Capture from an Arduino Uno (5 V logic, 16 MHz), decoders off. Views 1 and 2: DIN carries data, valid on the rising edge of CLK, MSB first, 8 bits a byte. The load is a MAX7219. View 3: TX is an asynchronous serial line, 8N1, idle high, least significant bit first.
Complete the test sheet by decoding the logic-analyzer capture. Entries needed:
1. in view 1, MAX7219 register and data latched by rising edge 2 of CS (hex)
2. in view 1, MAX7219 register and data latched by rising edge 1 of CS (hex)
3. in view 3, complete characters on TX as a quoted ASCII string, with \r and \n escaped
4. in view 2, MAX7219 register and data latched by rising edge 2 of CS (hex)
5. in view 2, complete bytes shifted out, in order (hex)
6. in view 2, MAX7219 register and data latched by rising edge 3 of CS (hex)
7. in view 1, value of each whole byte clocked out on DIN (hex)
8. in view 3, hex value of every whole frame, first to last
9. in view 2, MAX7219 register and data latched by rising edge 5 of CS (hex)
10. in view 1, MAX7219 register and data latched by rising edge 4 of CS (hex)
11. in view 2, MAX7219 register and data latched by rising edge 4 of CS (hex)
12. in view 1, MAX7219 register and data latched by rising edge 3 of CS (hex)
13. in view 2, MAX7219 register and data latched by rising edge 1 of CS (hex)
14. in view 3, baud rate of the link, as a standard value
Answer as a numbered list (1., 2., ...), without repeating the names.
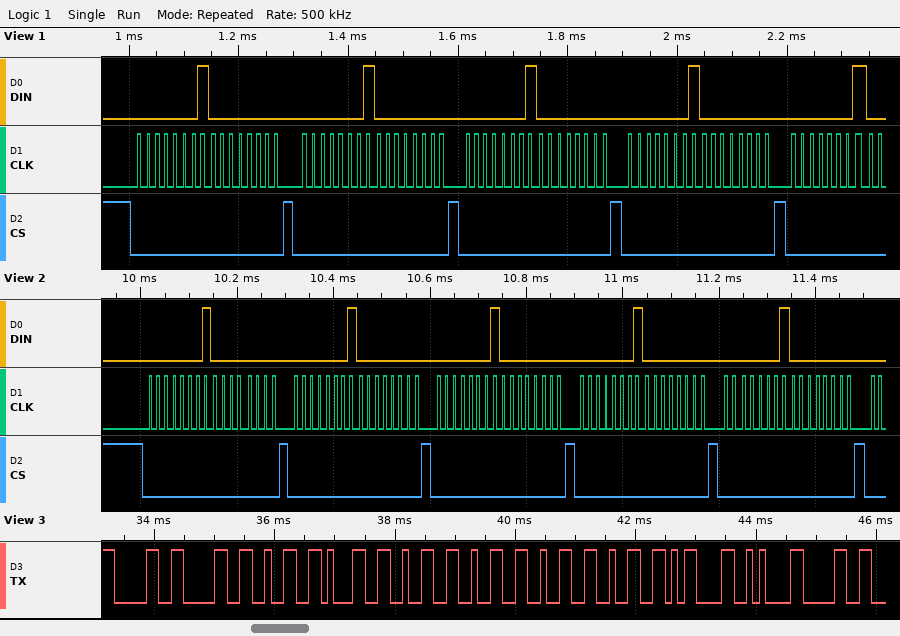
1. register 0x1, data 0x00
2. register 0x1, data 0x00
3. "00212222\r\n0"
4. register 0x1, data 0x00
5. 01 00 01 00 01 00 01 00 01 00
6. register 0x1, data 0x00
7. 01 00 01 00 01 00 01 00 01
8. 30 30 32 31 32 32 32 32 0D 0A 30
9. register 0x1, data 0x00
10. register 0x1, data 0x00
11. register 0x1, data 0x00
12. register 0x1, data 0x00
13. register 0x1, data 0x00
14. 9600 baud
